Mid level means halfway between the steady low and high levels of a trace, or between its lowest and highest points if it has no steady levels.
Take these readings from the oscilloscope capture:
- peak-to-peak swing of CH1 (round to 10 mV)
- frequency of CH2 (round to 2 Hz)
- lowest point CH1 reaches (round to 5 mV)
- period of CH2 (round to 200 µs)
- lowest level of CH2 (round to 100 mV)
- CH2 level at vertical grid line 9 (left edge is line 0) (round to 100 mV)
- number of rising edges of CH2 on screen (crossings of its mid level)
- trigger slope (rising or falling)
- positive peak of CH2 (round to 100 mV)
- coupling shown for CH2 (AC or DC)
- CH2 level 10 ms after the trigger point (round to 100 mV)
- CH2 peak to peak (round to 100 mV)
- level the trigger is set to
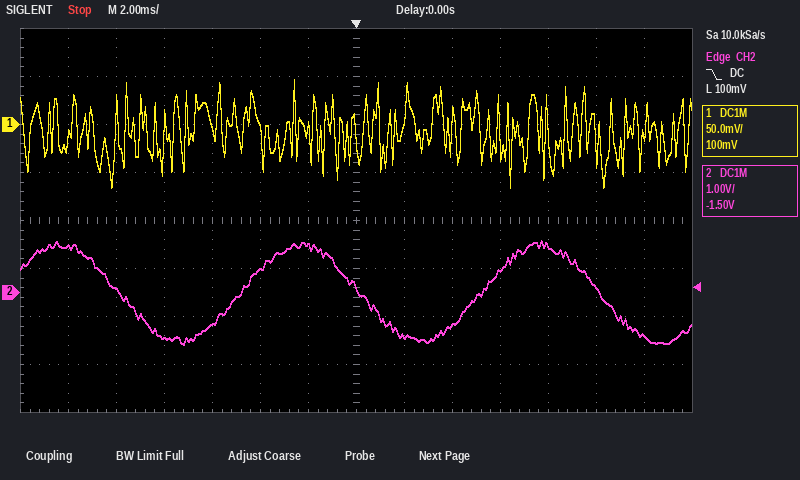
110 mV
100 Hz
-65 mV
10.0 ms
-1.1 V
-700 mV
2
falling
1.1 V
DC
100 mV
2.2 V
100 mV
